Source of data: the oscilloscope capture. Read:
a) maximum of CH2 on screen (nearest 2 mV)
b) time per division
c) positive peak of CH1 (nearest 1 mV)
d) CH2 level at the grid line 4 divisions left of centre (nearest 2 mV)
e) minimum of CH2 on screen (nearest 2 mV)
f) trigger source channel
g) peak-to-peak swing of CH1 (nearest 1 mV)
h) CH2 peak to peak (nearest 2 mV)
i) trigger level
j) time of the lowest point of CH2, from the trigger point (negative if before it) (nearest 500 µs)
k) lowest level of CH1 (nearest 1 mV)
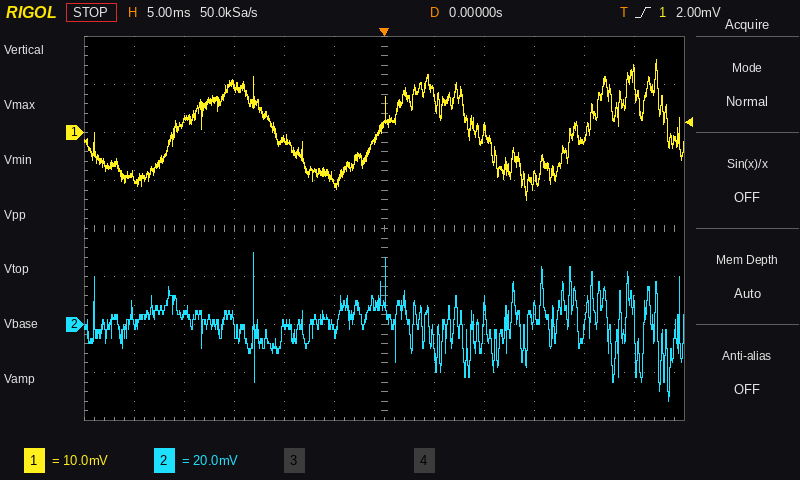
30 mV
5 ms
15 mV
4 mV
-32 mV
CH1
29 mV
62 mV
2.00 mV
+28.5 ms
-14 mV
